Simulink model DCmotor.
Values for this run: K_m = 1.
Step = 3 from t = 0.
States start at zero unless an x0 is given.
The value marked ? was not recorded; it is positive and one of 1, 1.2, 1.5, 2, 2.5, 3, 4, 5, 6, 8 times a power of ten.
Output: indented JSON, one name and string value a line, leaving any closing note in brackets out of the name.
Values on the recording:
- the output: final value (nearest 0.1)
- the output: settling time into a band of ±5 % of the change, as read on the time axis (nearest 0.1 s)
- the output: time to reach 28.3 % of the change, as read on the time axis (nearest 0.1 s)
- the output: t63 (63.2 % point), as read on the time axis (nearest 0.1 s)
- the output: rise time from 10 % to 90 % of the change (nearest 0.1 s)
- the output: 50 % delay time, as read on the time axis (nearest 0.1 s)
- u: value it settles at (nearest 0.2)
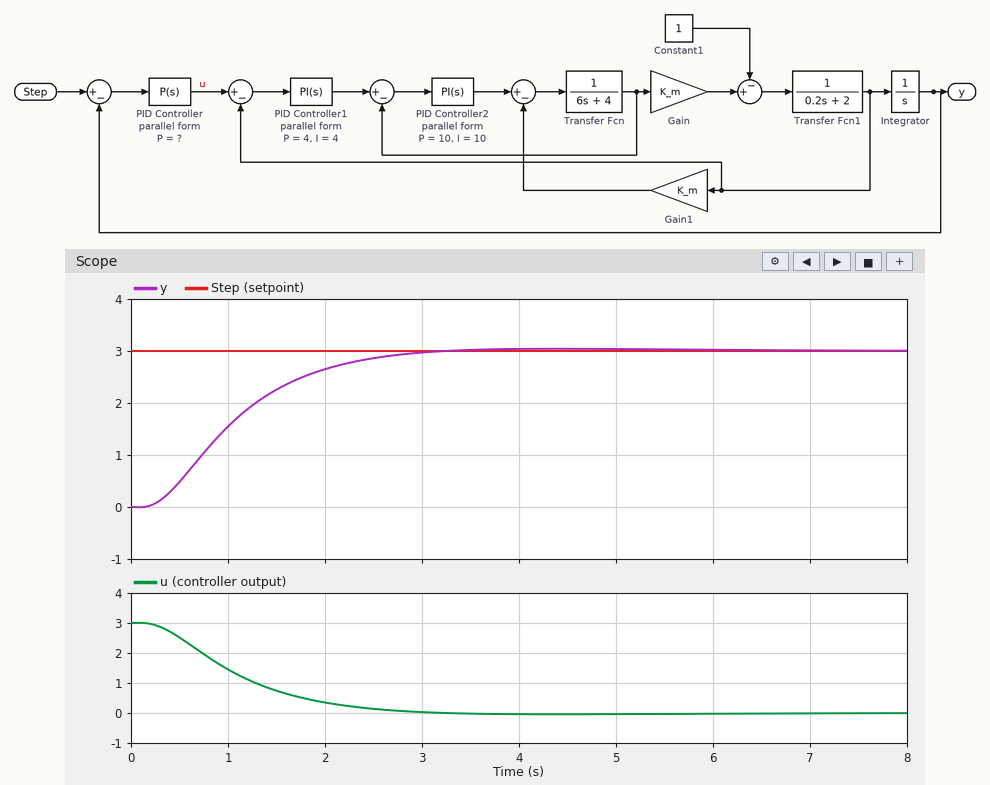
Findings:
{
  "the output: final value": "3.0",
  "the output: settling time into a band of ±5 % of the change, as read on the time axis": "2.5 s",
  "the output: time to reach 28.3 % of the change, as read on the time axis": "0.7 s",
  "the output: t63 (63.2 % point), as read on the time axis": "1.2 s",
  "the output: rise time from 10 % to 90 % of the change": "1.7 s",
  "the output: 50 % delay time, as read on the time axis": "1.0 s",
  "u: value it settles at": "0.0"
}
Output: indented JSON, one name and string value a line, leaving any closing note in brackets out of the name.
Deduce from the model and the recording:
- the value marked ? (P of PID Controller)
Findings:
{
  "the value marked ?": "1"
}
